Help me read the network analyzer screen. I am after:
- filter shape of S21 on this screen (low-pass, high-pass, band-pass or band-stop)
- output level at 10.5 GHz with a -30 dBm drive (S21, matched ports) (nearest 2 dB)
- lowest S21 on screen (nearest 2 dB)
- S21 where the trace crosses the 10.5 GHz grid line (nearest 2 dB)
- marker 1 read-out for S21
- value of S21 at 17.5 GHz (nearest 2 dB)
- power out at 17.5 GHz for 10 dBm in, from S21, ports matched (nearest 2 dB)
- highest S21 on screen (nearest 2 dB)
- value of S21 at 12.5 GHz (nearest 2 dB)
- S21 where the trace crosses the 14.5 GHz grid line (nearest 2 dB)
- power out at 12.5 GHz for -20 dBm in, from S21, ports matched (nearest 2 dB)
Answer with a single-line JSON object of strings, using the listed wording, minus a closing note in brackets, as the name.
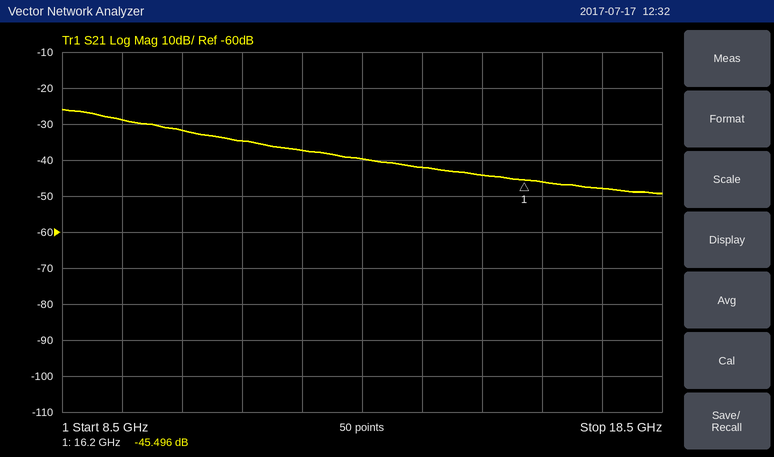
{"filter shape of S21 on this screen": "low-pass", "output level at 10.5 GHz with a -30 dBm drive (S21, matched ports)": "-62 dBm", "lowest S21 on screen": "-50 dB", "S21 where the trace crosses the 10.5 GHz grid line": "-32 dB", "marker 1 read-out for S21": "-45.496 dB", "value of S21 at 17.5 GHz": "-48 dB", "power out at 17.5 GHz for 10 dBm in, from S21, ports matched": "-38 dBm", "highest S21 on screen": "-26 dB", "value of S21 at 12.5 GHz": "-38 dB", "S21 where the trace crosses the 14.5 GHz grid line": "-42 dB", "power out at 12.5 GHz for -20 dBm in, from S21, ports matched": "-58 dBm"}
